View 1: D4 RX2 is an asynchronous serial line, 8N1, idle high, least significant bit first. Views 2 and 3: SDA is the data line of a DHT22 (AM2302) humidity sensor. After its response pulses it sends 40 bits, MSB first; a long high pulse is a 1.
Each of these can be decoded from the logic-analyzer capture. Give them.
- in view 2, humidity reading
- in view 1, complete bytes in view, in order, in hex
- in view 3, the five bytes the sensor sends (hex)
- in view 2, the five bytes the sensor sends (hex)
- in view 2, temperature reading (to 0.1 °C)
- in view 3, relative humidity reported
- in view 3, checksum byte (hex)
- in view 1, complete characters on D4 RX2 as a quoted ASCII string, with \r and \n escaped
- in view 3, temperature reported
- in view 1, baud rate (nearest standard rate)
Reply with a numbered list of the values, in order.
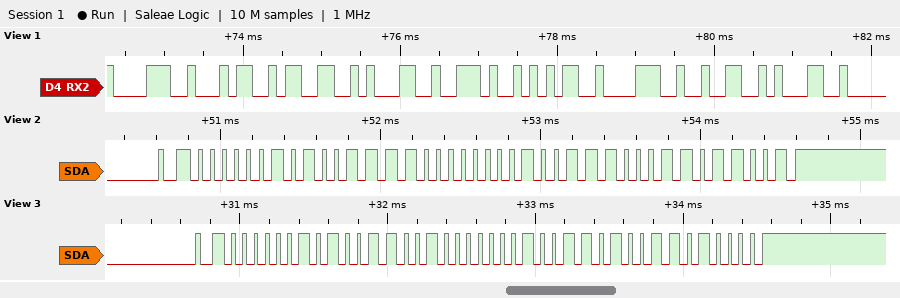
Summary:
1. 67.0 %
2. 38 34 33 31 2E 35 38 32 31
3. 02 99 01 34 D0
4. 02 9E 01 38 D9
5. 31.2 °C
6. 66.5 %
7. 0xD0
8. "8431.5821"
9. 30.8 °C
10. 9600 baud
